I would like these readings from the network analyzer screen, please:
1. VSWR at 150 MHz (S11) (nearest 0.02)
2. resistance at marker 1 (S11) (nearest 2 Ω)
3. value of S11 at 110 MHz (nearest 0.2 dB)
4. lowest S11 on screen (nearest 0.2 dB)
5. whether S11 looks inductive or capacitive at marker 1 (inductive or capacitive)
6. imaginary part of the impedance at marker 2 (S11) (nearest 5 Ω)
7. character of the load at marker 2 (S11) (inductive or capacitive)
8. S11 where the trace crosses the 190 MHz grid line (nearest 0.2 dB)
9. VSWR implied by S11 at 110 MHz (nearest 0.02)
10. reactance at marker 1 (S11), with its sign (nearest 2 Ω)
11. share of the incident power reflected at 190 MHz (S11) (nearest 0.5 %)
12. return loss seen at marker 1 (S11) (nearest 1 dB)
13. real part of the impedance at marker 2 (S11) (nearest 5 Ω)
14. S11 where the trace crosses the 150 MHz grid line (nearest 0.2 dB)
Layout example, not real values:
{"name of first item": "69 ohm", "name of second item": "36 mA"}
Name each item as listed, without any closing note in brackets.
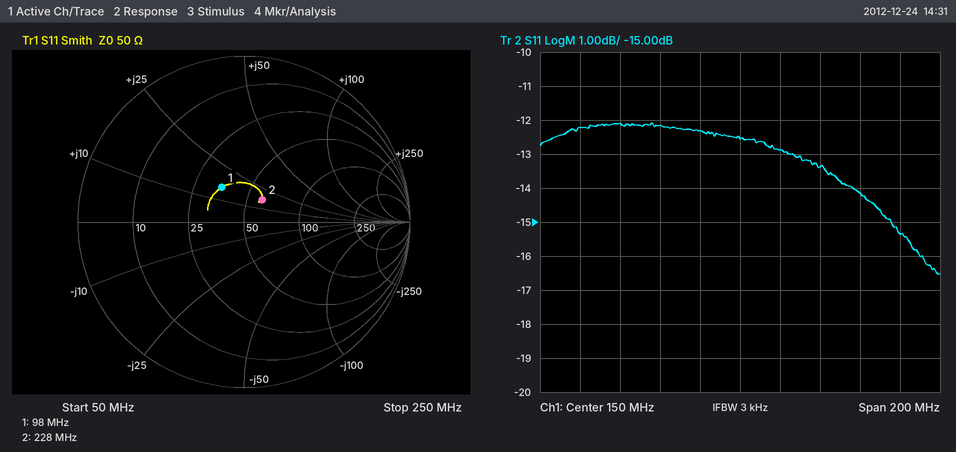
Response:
{"VSWR at 150 MHz (S11)": "1.62", "resistance at marker 1 (S11)": "36 Ω", "value of S11 at 110 MHz": "-12.2 dB", "lowest S11 on screen": "-16.6 dB", "whether S11 looks inductive or capacitive at marker 1": "inductive", "imaginary part of the impedance at marker 2 (S11)": "+15 Ω", "character of the load at marker 2 (S11)": "inductive", "S11 where the trace crosses the 190 MHz grid line": "-13.4 dB", "VSWR implied by S11 at 110 MHz": "1.66", "reactance at marker 1 (S11), with its sign": "+16 Ω", "share of the incident power reflected at 190 MHz (S11)": "4.5 %", "return loss seen at marker 1 (S11)": "12 dB", "real part of the impedance at marker 2 (S11)": "60 Ω", "S11 where the trace crosses the 150 MHz grid line": "-12.6 dB"}
